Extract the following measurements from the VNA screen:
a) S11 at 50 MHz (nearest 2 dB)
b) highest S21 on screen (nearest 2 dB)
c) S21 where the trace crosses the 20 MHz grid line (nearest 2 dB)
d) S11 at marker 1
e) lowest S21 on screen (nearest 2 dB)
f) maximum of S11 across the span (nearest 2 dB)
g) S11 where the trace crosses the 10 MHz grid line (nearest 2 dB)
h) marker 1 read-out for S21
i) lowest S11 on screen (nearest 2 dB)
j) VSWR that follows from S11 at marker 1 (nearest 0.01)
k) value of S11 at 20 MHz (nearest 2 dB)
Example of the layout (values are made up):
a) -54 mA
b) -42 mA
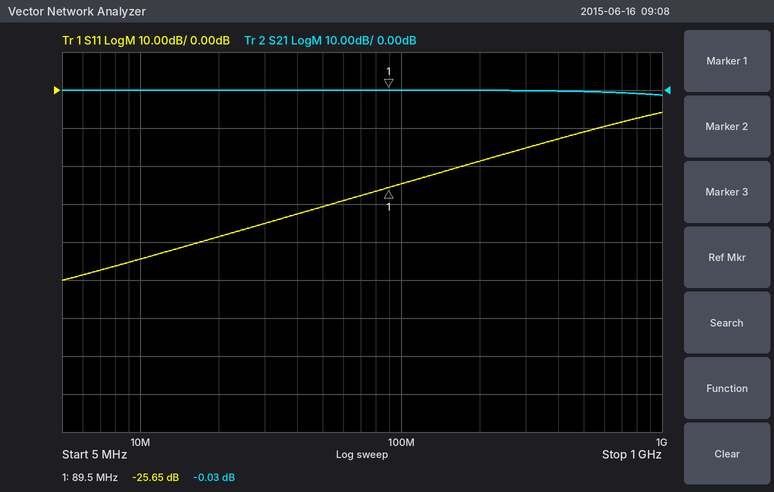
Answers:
a) -30 dB
b) 0 dB
c) 0 dB
d) -25.65 dB
e) -2 dB
f) -6 dB
g) -44 dB
h) -0.03 dB
i) -50 dB
j) 1.11
k) -38 dB
